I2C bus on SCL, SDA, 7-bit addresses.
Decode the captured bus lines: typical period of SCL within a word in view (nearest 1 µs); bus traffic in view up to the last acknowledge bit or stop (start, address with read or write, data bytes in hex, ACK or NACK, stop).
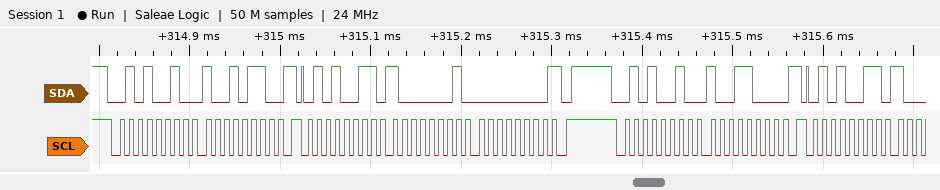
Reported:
10 µs
start, address 29 write ACK, 96 ACK, repeated start, address 29 read ACK, 81 ACK, 00 NACK, stop, start, address 29 write ACK, 98 ACK, repeated start, address 29 read ACK
